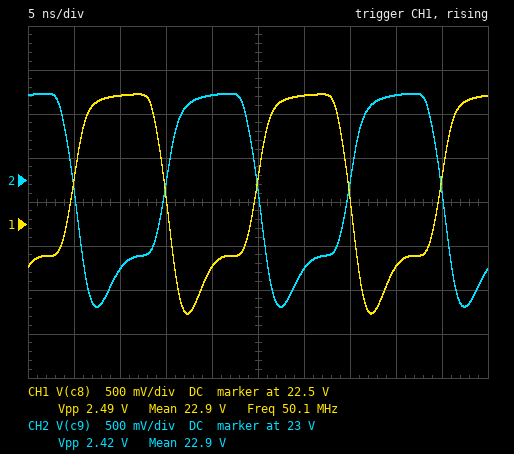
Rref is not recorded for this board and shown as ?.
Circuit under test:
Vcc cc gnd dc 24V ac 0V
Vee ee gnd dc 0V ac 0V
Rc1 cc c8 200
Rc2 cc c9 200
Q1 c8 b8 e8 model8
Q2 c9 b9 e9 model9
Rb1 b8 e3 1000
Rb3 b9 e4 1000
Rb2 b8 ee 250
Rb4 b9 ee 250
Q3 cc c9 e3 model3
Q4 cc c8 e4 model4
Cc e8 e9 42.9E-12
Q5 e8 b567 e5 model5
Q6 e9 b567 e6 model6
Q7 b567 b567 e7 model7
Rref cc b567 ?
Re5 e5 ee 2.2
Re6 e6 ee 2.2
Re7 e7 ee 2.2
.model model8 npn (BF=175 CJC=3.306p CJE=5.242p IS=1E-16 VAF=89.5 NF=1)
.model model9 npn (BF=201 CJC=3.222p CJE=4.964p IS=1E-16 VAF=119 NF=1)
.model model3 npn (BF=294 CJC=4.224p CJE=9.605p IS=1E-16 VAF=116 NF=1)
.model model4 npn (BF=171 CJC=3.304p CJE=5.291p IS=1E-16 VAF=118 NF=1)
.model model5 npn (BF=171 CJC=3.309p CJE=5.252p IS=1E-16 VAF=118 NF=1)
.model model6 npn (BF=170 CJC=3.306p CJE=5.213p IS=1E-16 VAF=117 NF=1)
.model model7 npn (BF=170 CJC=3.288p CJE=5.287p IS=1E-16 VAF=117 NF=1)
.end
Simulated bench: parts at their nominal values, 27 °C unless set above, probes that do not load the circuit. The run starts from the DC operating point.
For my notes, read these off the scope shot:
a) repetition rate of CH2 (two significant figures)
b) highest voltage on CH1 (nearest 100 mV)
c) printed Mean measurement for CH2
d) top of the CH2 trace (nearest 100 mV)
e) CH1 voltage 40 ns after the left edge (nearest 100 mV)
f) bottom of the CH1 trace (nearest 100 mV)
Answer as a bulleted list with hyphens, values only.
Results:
- 50 MHz
- 24.0 V
- 22.9 V
- 24.0 V
- 22.0 V
- 21.5 V
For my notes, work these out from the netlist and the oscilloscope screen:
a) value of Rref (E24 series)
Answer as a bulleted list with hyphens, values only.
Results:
- 4.3 kΩ
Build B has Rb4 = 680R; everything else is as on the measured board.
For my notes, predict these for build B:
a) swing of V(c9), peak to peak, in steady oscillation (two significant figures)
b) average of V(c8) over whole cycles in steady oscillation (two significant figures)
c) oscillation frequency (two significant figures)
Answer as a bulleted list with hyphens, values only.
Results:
- 2.8 V
- 23 V
- 35 MHz
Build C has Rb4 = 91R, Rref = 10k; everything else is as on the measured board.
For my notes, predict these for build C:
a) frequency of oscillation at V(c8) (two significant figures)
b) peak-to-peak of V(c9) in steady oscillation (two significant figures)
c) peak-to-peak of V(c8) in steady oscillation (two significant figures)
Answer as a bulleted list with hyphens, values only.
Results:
- 63 MHz
- 770 mV
- 820 mV
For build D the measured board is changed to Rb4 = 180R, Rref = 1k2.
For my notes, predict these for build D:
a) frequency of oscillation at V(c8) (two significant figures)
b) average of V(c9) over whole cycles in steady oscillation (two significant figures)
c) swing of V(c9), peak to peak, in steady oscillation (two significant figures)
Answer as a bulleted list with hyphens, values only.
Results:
- 57 MHz
- 20 V
- 8.7 V
